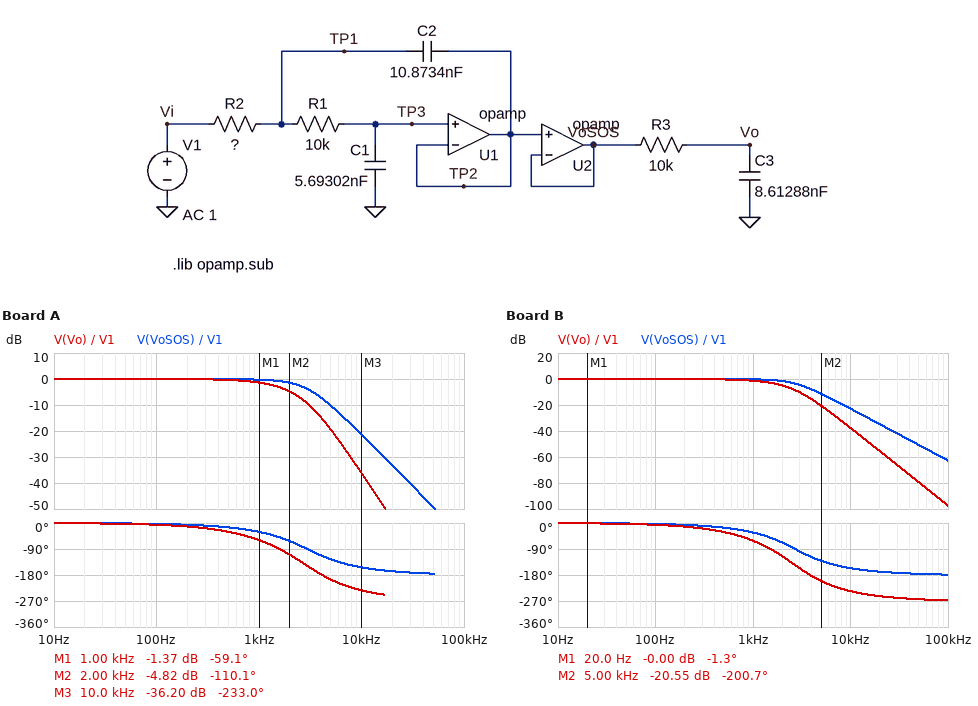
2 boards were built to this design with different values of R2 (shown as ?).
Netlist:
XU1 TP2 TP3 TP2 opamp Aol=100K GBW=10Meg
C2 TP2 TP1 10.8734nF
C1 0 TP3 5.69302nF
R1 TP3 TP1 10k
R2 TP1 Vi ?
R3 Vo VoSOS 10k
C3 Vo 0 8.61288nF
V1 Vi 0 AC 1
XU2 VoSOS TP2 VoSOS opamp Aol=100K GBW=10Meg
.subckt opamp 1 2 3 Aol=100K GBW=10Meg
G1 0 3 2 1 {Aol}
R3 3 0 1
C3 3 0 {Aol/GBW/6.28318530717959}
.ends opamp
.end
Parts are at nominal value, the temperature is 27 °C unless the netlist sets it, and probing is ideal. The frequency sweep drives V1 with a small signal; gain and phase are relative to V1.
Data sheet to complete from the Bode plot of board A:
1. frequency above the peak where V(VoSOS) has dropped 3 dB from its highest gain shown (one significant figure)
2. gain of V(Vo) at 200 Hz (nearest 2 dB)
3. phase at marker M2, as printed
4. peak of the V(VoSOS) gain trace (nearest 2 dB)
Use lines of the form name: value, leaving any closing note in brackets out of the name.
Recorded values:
frequency above the peak where V(VoSOS) has dropped 3 dB from its highest gain shown: 3 kHz
gain of V(Vo) at 200 Hz: 0 dB
phase at marker M2, as printed: -110.1 deg
peak of the V(VoSOS) gain trace: 0 dB
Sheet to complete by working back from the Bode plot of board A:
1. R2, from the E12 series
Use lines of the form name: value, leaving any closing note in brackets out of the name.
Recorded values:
R2, from the E12 series: 4.7 kΩ
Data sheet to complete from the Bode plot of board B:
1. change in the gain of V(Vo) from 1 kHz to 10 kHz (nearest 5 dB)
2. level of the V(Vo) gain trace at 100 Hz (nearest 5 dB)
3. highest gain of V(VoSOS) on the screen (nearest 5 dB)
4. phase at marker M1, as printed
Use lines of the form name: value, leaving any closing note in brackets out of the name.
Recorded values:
change in the gain of V(Vo) from 1 kHz to 10 kHz: -35 dB
level of the V(Vo) gain trace at 100 Hz: 0 dB
highest gain of V(VoSOS) on the screen: 0 dB
phase at marker M1, as printed: -1.3 deg
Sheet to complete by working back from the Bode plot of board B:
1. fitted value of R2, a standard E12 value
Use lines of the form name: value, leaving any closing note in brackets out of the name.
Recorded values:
fitted value of R2, a standard E12 value: 5.6 kΩ
